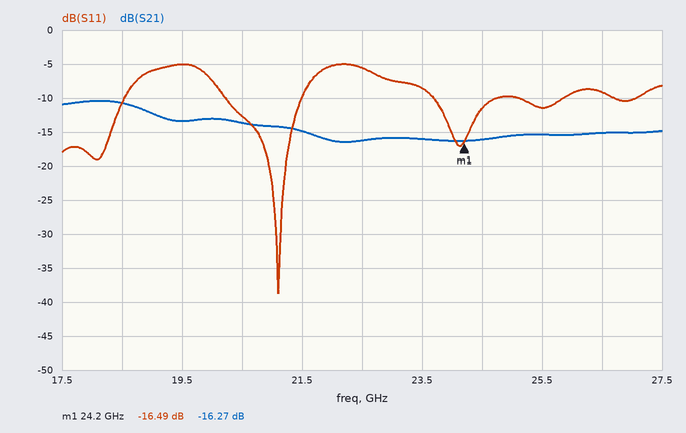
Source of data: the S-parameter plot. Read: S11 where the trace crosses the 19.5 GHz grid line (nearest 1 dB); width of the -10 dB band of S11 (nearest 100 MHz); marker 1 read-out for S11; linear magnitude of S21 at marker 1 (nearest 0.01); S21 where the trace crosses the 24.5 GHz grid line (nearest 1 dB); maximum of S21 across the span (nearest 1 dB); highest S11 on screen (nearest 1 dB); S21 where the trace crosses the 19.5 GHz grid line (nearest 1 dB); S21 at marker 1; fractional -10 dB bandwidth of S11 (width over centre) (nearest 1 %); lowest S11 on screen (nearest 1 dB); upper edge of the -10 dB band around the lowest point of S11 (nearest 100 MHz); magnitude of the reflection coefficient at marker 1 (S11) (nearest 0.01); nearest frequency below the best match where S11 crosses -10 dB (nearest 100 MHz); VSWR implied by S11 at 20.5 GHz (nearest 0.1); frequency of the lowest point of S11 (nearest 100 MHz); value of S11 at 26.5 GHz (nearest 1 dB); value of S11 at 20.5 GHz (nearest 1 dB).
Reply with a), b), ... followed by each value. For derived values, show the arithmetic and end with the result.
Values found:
a) -5 dB
b) 21.5 GHz − 20.2 GHz = 1.3 GHz
c) -16.49 dB
d) 10^(-16.27/20) ≈ 0.15
e) -16 dB
f) -10 dB
g) -5 dB
h) -13 dB
i) -16.27 dB
j) 1.3 GHz / 20.85 GHz ≈ 6 %
k) -39 dB
l) 21.5 GHz
m) 10^(-16.49/20) ≈ 0.15
n) 20.2 GHz
o) |Γ| = 10^(-13/20) = 0.2239; VSWR = (1 + 0.2239)/(1 − 0.2239) ≈ 1.6
p) 21.1 GHz
q) -9 dB
r) -13 dB
